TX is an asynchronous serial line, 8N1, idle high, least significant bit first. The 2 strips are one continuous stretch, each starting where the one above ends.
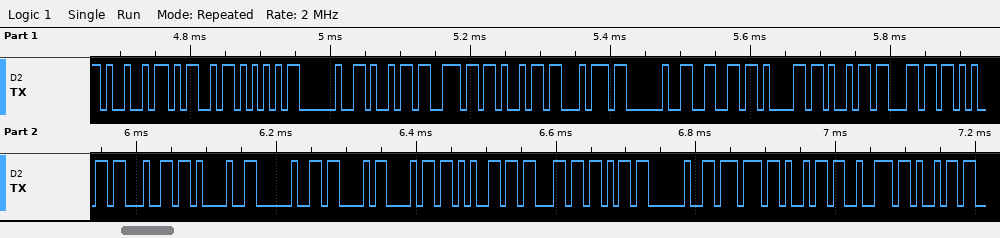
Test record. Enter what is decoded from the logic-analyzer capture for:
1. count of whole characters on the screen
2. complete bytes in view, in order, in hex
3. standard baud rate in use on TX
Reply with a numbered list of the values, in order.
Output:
1. 27
2. 0x49 0x4D 0x55 0x20 0x69 0x6E 0x69 0x74 0x20 0x66 0x61 0x69 0x6C 0x65 0x64 0x21 0x20 0x43 0x68 0x65 0x63 0x6B 0x20 0x77 0x69 0x72 0x69
3. 115200 baud
